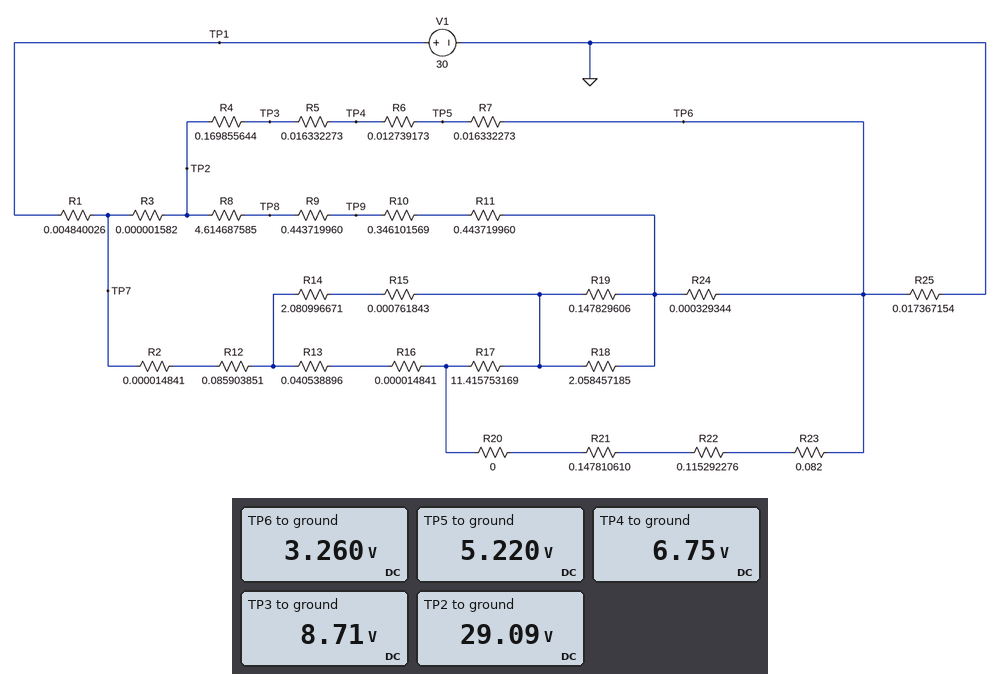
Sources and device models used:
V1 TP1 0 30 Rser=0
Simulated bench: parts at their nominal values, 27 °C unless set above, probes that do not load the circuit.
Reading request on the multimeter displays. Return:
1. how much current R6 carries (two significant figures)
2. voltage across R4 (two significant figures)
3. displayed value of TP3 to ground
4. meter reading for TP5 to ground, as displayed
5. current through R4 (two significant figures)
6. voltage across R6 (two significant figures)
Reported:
120 A
20 V
8.71 V
5.220 V
120 A
1.5 V
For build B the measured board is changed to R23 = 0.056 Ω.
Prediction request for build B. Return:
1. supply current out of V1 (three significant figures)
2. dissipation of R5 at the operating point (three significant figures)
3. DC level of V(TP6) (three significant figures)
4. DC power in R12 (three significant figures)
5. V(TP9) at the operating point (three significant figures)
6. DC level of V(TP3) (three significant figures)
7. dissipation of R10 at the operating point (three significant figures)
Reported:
190 A
234 W
3.30 V
375 W
6.79 V
8.74 V
6.72 W
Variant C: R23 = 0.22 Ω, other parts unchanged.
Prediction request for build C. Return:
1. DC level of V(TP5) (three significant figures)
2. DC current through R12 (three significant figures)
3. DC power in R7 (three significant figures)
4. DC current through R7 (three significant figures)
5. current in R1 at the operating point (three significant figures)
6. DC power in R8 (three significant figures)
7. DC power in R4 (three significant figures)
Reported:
5.06 V
52.3 A
239 W
121 A
178 A
91.5 W
2.49 kW
